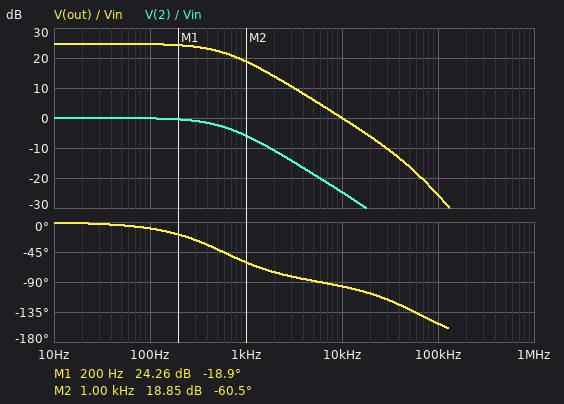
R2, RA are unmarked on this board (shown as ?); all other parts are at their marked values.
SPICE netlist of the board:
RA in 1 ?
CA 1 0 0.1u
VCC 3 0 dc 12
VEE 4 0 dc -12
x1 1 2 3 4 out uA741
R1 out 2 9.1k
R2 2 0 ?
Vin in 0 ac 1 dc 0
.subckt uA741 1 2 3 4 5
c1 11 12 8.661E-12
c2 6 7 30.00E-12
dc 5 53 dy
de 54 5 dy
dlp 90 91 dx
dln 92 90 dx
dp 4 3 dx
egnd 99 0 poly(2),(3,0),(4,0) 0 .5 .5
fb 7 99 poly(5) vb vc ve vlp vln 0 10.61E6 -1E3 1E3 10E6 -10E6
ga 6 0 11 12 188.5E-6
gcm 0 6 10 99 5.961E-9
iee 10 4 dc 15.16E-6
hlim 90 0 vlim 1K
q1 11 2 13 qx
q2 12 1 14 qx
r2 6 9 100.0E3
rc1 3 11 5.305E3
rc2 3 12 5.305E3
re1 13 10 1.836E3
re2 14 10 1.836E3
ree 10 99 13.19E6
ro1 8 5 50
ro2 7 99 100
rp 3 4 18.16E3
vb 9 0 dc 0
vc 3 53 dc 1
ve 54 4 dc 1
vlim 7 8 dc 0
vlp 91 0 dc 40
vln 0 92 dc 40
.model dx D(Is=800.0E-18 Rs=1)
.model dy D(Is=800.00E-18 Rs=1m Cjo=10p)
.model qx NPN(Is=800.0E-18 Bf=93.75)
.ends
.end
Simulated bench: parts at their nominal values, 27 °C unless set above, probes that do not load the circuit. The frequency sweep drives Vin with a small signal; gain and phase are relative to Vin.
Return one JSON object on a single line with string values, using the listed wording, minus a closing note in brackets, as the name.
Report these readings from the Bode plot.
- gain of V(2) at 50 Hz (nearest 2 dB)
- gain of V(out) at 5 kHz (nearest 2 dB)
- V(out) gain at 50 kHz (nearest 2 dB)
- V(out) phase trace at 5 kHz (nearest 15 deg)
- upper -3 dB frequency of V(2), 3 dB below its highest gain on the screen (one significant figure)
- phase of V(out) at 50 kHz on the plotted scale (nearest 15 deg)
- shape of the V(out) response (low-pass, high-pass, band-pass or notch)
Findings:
{"gain of V(2) at 50 Hz": "0 dB", "gain of V(out) at 5 kHz": "6 dB", "V(out) gain at 50 kHz": "-16 dB", "V(out) phase trace at 5 kHz": "-90 deg", "upper -3 dB frequency of V(2), 3 dB below its highest gain on the screen": "600 Hz", "phase of V(out) at 50 kHz on the plotted scale": "-135 deg", "shape of the V(out) response": "low-pass"}
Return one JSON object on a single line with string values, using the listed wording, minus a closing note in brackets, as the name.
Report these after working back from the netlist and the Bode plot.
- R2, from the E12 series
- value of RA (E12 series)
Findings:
{"R2, from the E12 series": "560 Ω", "value of RA": "2.7 kΩ"}
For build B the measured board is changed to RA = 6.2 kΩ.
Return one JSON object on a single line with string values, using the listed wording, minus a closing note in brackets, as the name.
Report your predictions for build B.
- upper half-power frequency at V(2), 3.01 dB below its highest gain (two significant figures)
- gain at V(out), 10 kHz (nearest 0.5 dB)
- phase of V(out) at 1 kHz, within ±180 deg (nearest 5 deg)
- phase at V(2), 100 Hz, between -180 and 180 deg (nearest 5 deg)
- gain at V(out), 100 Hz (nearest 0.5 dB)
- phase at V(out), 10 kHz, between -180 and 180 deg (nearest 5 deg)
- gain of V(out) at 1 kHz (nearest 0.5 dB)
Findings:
{"upper half-power frequency at V(2), 3.01 dB below its highest gain": "260 Hz", "gain at V(out), 10 kHz": "-7.0 dB", "phase of V(out) at 1 kHz, within ±180 deg": "-75 deg", "phase at V(2), 100 Hz, between -180 and 180 deg": "-20 deg", "gain at V(out), 100 Hz": "24.0 dB", "phase at V(out), 10 kHz, between -180 and 180 deg": "-100 deg", "gain of V(out) at 1 kHz": "12.5 dB"}
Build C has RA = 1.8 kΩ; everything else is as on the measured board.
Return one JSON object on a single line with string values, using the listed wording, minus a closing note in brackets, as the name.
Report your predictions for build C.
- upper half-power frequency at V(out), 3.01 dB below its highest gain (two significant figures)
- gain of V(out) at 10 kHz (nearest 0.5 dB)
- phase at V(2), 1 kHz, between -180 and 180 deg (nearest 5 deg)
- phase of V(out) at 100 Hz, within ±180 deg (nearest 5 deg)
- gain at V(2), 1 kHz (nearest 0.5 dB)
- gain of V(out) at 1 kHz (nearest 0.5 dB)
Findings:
{"upper half-power frequency at V(out), 3.01 dB below its highest gain": "880 Hz", "gain of V(out) at 10 kHz": "3.5 dB", "phase at V(2), 1 kHz, between -180 and 180 deg": "-50 deg", "phase of V(out) at 100 Hz, within ±180 deg": "-5 deg", "gain at V(2), 1 kHz": "-3.5 dB", "gain of V(out) at 1 kHz": "21.0 dB"}
